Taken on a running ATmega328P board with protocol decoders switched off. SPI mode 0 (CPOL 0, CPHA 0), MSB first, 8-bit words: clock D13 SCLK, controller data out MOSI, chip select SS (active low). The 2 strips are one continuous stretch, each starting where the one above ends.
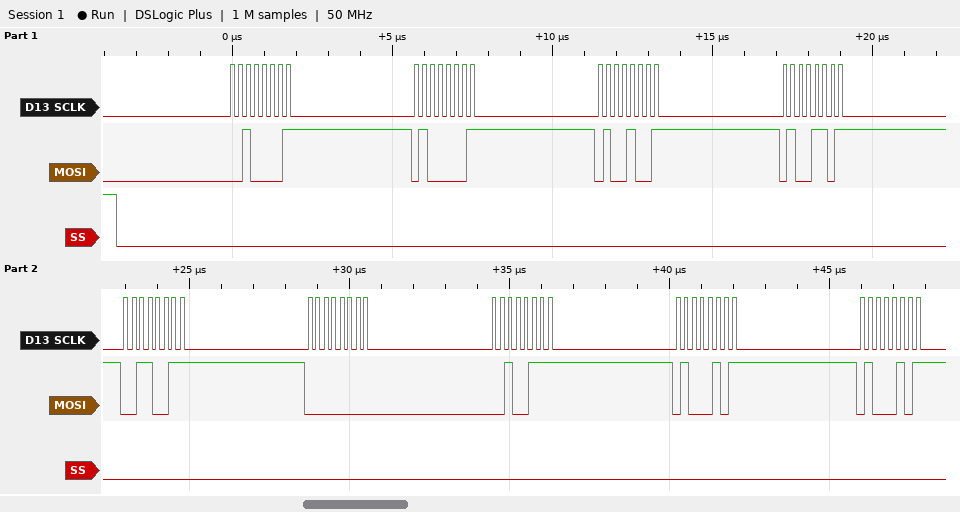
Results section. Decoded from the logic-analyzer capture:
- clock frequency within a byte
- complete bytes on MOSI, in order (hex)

4 MHz
0x21 0x41 0x49 0x4D 0x33 0x00 0x27 0x45 0x45
